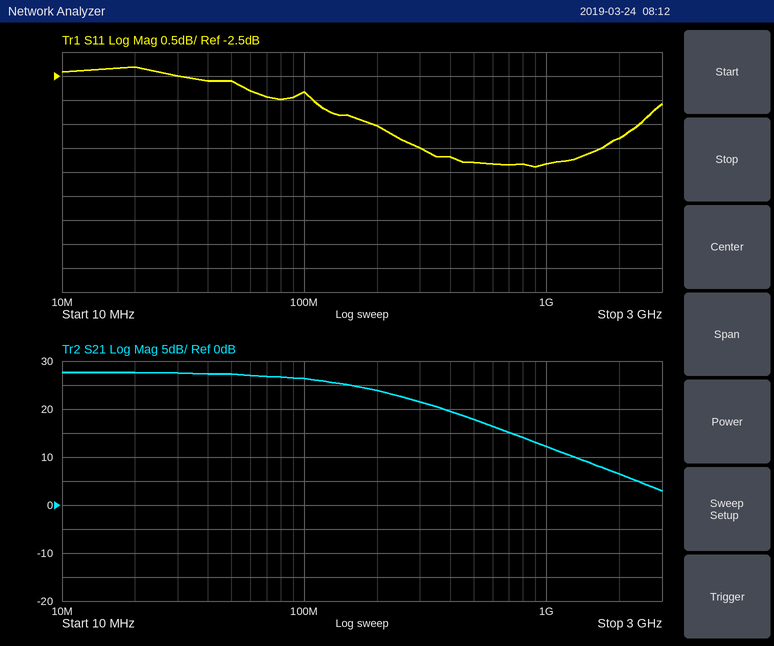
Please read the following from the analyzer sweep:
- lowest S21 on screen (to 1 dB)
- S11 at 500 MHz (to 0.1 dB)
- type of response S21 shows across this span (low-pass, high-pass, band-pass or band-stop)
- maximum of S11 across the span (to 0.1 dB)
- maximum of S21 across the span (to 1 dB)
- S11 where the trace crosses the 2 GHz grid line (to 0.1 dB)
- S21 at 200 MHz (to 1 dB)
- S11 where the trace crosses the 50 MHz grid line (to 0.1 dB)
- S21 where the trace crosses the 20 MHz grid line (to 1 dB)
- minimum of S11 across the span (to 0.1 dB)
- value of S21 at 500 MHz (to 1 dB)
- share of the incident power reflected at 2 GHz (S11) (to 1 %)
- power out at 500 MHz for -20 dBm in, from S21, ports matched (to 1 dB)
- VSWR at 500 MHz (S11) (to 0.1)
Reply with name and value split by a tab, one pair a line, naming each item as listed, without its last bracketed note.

lowest S21 on screen	3 dB
S11 at 500 MHz	-4.3 dB
type of response S21 shows across this span	low-pass
maximum of S11 across the span	-2.3 dB
maximum of S21 across the span	28 dB
S11 where the trace crosses the 2 GHz grid line	-3.8 dB
S21 at 200 MHz	24 dB
S11 where the trace crosses the 50 MHz grid line	-2.6 dB
S21 where the trace crosses the 20 MHz grid line	28 dB
minimum of S11 across the span	-4.4 dB
value of S21 at 500 MHz	18 dB
share of the incident power reflected at 2 GHz (S11)	42 %
power out at 500 MHz for -20 dBm in, from S21, ports matched	-2 dBm
VSWR at 500 MHz (S11)	4.1
